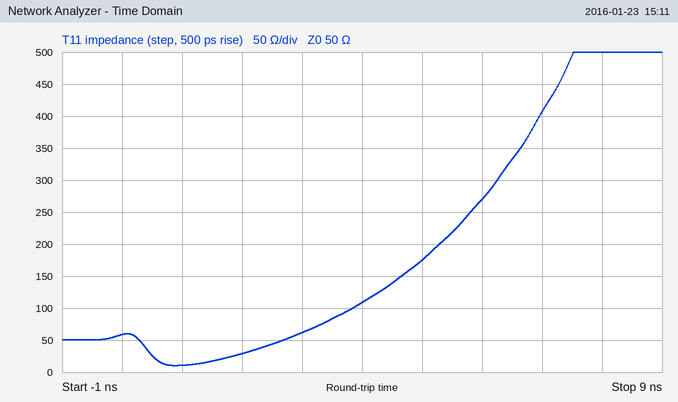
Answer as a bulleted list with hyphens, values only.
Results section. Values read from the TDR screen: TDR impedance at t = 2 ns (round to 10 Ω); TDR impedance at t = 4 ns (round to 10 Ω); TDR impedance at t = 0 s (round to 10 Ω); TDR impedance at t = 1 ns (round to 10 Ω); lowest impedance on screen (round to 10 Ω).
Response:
- 30 Ω
- 110 Ω
- 60 Ω
- 10 Ω
- 10 Ω
